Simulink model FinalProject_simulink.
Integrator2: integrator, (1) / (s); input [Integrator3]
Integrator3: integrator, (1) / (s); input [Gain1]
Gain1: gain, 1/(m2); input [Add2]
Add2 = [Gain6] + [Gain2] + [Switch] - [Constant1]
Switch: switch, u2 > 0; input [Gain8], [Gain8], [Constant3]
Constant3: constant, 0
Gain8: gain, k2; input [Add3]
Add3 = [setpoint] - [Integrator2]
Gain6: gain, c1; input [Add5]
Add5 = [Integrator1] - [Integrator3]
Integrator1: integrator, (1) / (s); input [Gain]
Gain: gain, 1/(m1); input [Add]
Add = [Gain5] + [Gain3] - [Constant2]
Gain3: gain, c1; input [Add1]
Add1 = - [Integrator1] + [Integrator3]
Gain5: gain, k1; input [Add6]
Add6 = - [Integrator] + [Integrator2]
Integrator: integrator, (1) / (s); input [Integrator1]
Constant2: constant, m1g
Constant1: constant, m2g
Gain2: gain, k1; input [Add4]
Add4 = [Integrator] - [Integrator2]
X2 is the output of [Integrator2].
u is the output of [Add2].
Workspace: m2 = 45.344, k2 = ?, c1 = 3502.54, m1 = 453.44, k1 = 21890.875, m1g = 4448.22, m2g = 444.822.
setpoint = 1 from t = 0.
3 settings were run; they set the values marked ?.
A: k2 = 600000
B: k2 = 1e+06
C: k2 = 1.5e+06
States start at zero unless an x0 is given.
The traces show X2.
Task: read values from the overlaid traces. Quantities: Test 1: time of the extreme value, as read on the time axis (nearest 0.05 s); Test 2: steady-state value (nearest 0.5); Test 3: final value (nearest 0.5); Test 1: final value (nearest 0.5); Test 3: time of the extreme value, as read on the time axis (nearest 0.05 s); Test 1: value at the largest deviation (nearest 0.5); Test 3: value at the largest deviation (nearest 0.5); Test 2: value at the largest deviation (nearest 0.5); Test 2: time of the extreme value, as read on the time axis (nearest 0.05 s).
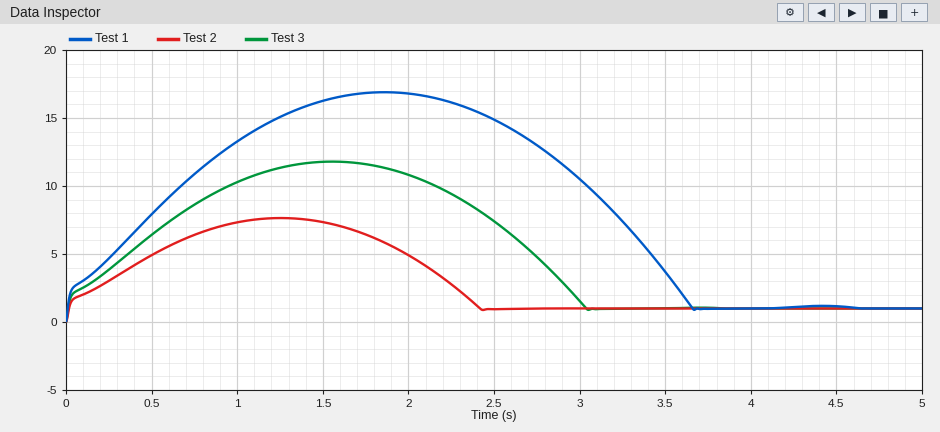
1.85 s
1.0
1.0
1.0
1.55 s
17.0
12.0
7.5
1.25 s
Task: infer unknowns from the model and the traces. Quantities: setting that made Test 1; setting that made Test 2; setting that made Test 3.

C
A
B
